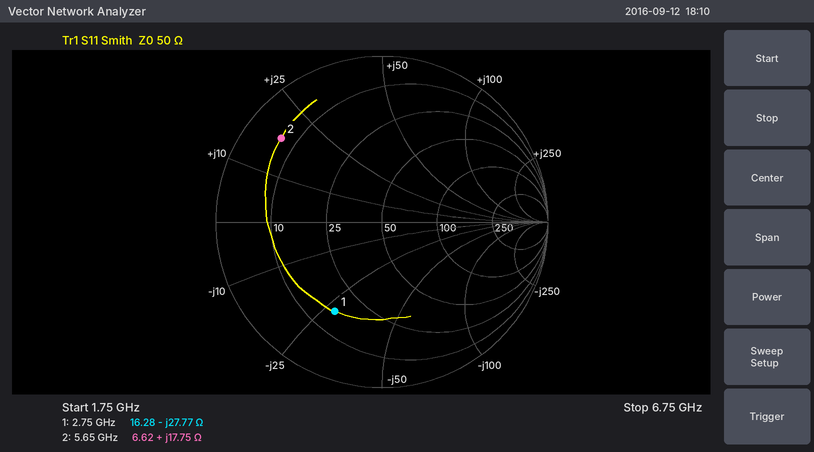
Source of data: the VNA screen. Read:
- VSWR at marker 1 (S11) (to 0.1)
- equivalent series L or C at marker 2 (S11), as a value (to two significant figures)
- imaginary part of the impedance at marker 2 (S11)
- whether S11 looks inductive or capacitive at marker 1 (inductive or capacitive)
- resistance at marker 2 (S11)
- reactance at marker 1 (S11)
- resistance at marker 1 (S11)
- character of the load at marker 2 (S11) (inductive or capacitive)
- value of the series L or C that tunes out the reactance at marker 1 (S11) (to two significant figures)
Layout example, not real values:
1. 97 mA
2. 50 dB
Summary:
1. 4.1
2. 500 pH
3. +17.75 Ω
4. capacitive
5. 6.62 Ω
6. -27.77 Ω
7. 16.28 Ω
8. inductive
9. 1.6 nH
